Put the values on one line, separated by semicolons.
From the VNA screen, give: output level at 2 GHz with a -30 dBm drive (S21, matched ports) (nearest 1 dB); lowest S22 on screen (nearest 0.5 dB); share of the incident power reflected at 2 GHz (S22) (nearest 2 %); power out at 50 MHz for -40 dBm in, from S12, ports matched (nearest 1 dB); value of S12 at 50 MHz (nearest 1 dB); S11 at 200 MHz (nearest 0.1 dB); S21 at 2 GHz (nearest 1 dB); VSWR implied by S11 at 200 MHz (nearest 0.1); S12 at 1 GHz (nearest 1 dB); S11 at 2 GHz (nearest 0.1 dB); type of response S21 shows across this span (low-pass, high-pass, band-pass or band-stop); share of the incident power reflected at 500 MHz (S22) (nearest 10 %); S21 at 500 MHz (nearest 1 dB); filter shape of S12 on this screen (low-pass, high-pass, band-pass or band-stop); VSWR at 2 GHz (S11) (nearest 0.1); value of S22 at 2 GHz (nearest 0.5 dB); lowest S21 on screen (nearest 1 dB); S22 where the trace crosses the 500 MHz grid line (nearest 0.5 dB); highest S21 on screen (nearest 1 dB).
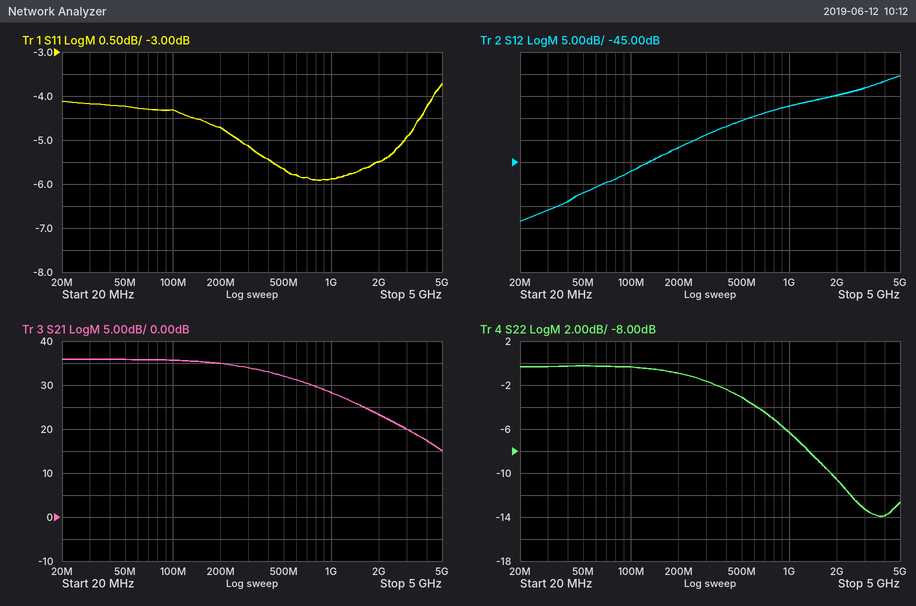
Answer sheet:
-7 dBm; -14.0 dB; 8 %; -92 dBm; -52 dB; -4.7 dB; 23 dB; 3.8; -32 dB; -5.5 dB; low-pass; 50 %; 32 dB; high-pass; 3.3; -10.5 dB; 15 dB; -3.0 dB; 36 dB
